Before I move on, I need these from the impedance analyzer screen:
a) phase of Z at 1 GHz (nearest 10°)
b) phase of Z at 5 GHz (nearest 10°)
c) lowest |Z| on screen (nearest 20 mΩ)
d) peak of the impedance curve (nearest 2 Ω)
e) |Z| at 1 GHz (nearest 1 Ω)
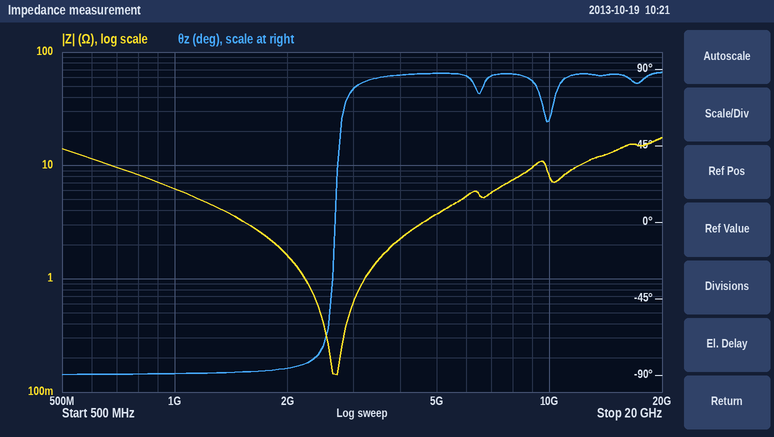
-90°
90°
140 mΩ
18 Ω
6 Ω
